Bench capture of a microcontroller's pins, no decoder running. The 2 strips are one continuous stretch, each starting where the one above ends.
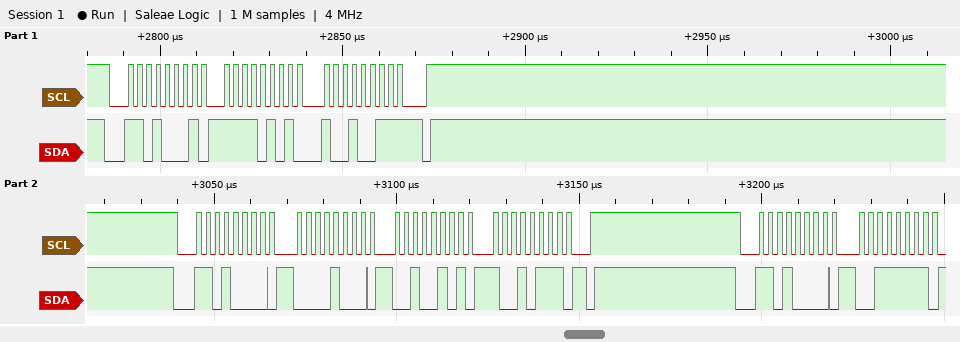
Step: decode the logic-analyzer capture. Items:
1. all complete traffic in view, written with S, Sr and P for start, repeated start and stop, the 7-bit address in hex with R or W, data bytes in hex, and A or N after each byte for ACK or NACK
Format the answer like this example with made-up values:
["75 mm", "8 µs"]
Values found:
["S 68R A F5 A 93 N P S 68W A 08 A 25 A 97 A P S 68W A 3F A"]
